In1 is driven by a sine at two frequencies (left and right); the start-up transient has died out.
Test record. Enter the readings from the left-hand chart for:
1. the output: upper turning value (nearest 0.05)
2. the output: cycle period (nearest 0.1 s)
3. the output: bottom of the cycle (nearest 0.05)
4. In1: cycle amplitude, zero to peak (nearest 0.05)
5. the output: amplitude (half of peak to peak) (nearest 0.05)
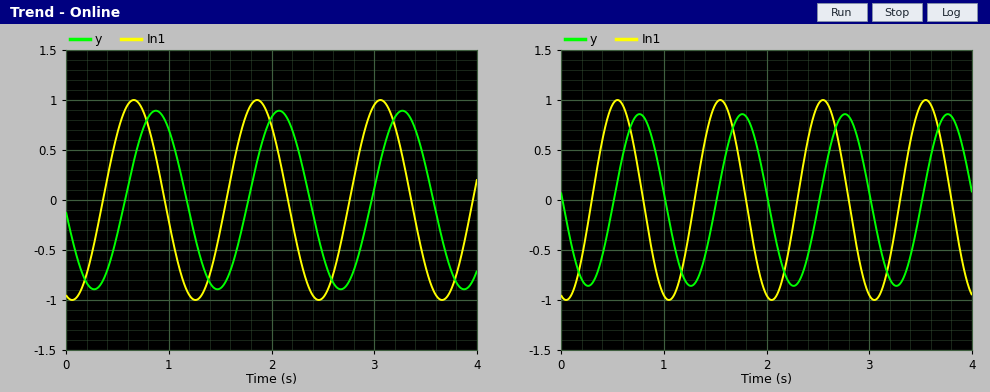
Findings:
0.90
1.2 s
-0.90
1.00
0.90
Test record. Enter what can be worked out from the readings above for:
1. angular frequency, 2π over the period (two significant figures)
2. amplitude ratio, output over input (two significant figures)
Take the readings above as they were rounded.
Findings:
5.2 rad/s
0.90
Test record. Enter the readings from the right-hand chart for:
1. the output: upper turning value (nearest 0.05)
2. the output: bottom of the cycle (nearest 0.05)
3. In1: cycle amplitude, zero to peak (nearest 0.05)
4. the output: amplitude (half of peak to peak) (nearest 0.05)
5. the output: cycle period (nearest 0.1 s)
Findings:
0.85
-0.85
1.00
0.85
1.0 s
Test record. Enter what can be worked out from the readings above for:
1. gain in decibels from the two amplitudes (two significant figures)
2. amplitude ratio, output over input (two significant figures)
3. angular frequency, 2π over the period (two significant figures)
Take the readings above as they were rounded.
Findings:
-1.4 dB
0.85
6.3 rad/s
